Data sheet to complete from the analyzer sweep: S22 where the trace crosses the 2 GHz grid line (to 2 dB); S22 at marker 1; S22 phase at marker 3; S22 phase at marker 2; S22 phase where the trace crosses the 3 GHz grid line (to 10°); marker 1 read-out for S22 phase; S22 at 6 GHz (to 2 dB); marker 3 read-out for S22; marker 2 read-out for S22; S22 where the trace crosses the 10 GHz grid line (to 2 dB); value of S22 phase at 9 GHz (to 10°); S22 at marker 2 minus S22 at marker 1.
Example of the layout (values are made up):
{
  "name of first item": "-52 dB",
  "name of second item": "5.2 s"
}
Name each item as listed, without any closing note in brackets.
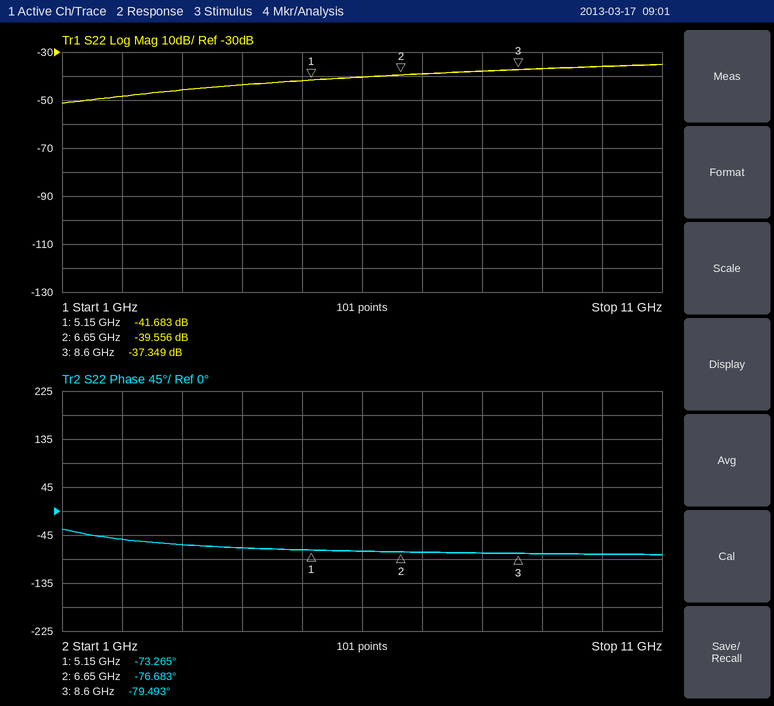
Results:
{
  "S22 where the trace crosses the 2 GHz grid line": "-48 dB",
  "S22 at marker 1": "-41.683 dB",
  "S22 phase at marker 3": "-79.493°",
  "S22 phase at marker 2": "-76.683°",
  "S22 phase where the trace crosses the 3 GHz grid line": "-60°",
  "marker 1 read-out for S22 phase": "-73.265°",
  "S22 at 6 GHz": "-40 dB",
  "marker 3 read-out for S22": "-37.349 dB",
  "marker 2 read-out for S22": "-39.556 dB",
  "S22 where the trace crosses the 10 GHz grid line": "-36 dB",
  "value of S22 phase at 9 GHz": "-80°",
  "S22 at marker 2 minus S22 at marker 1": "2.127 dB"
}
